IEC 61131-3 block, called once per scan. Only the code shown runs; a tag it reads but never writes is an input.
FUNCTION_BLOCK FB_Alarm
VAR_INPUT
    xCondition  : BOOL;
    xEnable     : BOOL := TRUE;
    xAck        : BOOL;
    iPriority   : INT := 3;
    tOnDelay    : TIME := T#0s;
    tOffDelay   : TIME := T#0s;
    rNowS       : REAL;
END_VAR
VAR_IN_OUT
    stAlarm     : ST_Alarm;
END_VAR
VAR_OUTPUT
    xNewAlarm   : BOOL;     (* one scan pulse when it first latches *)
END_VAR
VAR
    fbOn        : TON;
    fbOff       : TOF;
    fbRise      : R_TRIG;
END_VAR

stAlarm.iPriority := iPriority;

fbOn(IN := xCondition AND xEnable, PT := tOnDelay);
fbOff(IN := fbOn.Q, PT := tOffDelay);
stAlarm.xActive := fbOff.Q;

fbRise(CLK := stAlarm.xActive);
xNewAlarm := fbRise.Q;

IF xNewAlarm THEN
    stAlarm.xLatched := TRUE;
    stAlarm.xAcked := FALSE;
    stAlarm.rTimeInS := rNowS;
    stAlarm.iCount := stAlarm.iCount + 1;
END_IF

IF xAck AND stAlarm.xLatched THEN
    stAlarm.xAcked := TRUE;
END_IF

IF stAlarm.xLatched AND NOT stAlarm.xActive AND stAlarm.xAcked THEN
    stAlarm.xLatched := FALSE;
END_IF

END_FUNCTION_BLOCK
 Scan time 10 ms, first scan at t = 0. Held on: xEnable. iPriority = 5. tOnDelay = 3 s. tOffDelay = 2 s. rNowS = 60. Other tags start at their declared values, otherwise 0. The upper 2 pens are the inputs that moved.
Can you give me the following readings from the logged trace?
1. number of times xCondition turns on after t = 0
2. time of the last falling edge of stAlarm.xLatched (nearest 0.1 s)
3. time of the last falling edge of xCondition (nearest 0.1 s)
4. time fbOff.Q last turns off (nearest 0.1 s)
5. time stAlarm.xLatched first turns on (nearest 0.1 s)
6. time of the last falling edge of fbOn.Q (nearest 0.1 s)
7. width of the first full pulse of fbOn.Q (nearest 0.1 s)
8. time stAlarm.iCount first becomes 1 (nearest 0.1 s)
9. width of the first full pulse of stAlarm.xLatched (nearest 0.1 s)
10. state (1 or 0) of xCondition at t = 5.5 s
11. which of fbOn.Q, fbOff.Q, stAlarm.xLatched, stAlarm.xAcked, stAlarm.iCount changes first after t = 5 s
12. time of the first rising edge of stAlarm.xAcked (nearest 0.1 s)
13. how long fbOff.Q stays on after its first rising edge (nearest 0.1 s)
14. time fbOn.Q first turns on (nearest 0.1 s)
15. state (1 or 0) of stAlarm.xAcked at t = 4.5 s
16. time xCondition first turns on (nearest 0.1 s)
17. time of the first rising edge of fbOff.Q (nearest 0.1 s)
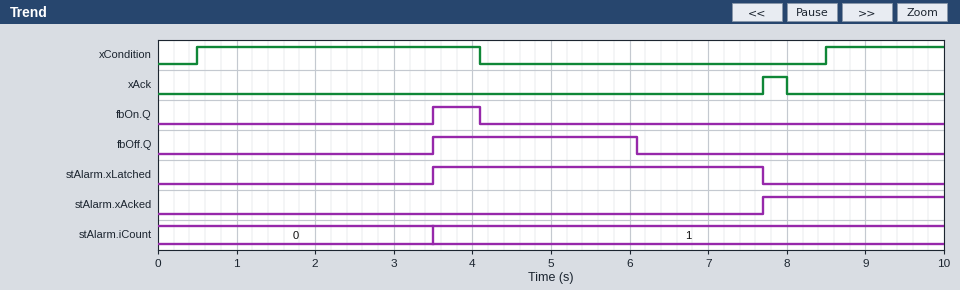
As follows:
2
7.7 s
4.1 s
6.1 s
3.5 s
4.1 s
0.6 s
3.5 s
4.2 s
0
fbOff.Q
7.7 s
2.6 s
3.5 s
0
0.5 s
3.5 s
